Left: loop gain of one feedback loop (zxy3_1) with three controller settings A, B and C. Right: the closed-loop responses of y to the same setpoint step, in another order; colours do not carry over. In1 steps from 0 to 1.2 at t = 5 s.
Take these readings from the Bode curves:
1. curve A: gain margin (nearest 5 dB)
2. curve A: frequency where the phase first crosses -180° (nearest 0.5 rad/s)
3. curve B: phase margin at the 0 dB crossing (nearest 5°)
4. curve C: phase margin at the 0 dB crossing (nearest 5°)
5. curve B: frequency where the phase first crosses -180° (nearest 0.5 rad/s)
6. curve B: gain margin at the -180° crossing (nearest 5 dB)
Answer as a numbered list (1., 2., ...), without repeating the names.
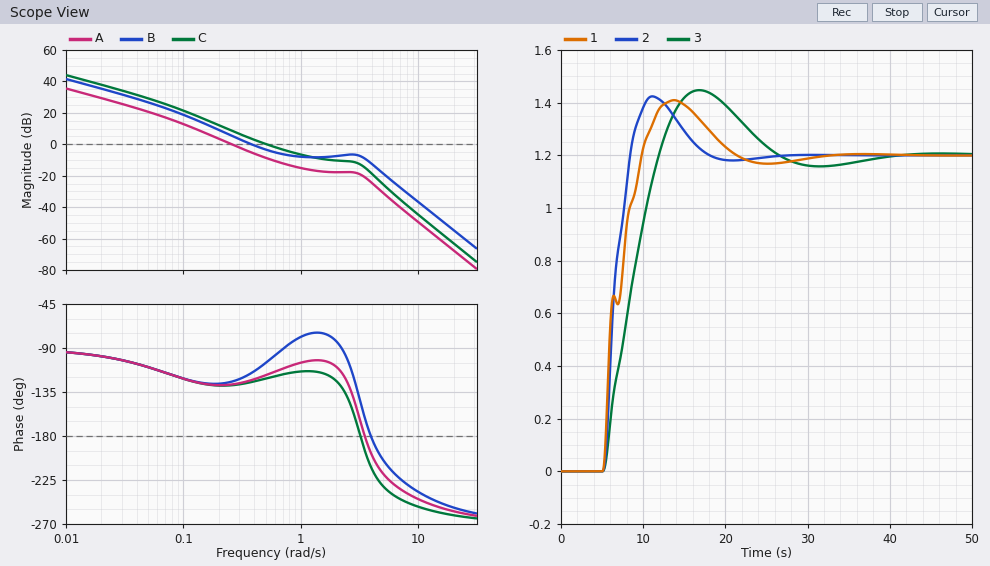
1. 20 dB
2. 3.5 rad/s
3. 65°
4. 60°
5. 4.0 rad/s
6. 10 dB
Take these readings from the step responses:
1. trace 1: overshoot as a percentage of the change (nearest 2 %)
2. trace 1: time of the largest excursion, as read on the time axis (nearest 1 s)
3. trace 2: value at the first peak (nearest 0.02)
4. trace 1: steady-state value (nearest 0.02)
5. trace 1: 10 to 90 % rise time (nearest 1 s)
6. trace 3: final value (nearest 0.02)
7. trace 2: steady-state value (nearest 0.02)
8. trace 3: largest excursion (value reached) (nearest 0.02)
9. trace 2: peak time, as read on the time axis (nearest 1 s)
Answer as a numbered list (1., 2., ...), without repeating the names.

1. 18 %
2. 14 s
3. 1.42
4. 1.20
5. 4 s
6. 1.20
7. 1.20
8. 1.44
9. 11 s
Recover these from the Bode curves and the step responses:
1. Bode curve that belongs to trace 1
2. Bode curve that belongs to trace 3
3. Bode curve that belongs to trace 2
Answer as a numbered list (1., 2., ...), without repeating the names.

1. B
2. A
3. C
